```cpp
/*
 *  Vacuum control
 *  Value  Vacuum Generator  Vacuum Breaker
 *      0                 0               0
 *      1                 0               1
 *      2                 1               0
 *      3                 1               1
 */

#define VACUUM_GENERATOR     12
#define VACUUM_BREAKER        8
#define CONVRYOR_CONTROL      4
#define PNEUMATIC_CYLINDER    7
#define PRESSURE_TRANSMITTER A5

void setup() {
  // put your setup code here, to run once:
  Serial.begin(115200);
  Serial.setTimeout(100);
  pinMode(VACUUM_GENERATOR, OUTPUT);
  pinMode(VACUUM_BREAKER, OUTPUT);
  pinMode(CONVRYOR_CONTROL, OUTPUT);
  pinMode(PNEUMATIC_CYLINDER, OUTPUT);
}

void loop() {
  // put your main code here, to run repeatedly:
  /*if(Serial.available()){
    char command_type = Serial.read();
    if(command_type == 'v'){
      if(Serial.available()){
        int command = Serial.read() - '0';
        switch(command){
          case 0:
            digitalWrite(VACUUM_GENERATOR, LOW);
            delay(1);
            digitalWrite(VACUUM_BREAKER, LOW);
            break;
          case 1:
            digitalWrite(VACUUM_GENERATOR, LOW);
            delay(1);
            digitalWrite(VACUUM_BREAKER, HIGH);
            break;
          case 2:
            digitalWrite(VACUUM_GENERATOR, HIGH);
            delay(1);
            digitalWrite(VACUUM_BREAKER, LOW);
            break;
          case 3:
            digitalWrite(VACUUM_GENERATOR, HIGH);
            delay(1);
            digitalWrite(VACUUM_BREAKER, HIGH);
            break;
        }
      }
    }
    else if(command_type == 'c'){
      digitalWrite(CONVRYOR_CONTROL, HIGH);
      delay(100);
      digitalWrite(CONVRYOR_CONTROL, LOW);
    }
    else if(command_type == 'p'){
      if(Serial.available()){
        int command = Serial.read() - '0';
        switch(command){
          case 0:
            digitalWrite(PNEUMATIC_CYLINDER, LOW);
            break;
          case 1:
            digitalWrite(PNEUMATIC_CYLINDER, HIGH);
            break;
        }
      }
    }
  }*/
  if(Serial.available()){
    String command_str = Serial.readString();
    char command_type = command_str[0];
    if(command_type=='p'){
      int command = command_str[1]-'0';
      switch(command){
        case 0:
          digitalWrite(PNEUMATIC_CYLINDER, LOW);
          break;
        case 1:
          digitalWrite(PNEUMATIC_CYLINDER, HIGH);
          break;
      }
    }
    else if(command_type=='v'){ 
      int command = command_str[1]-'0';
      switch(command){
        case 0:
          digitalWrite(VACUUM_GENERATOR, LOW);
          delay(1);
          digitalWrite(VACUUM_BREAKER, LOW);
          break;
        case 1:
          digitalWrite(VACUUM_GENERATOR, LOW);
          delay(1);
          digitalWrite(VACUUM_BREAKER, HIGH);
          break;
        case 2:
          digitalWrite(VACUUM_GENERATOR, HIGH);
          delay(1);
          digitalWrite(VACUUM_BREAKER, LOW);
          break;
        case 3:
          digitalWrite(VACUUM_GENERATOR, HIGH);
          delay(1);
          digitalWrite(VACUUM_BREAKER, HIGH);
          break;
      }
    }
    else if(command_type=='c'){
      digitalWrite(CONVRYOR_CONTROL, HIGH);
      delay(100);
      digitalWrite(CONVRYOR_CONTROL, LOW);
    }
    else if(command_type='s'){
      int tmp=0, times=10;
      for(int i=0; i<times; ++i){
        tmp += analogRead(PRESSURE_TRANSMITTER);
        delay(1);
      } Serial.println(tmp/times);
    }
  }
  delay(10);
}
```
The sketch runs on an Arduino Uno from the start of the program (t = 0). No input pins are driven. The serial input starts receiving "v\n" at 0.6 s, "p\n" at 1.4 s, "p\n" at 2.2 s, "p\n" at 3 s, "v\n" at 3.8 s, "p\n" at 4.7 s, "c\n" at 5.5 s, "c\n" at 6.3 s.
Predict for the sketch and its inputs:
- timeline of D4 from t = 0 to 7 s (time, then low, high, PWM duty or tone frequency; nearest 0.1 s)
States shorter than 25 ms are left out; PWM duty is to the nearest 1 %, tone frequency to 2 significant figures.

0 s low; 5.6 s high; 5.7 s low; 6.4 s high; 6.5 s low
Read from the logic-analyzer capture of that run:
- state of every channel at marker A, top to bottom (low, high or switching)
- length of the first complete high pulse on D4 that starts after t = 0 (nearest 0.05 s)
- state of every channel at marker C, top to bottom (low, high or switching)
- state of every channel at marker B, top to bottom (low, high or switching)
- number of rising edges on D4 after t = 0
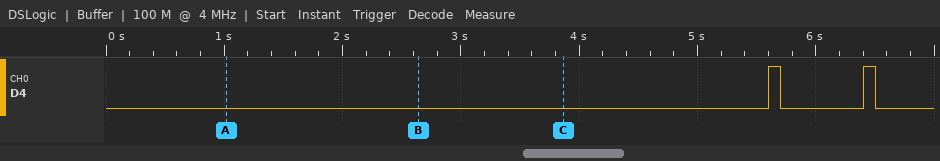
D4 low
0.10 s
D4 low
D4 low
2
